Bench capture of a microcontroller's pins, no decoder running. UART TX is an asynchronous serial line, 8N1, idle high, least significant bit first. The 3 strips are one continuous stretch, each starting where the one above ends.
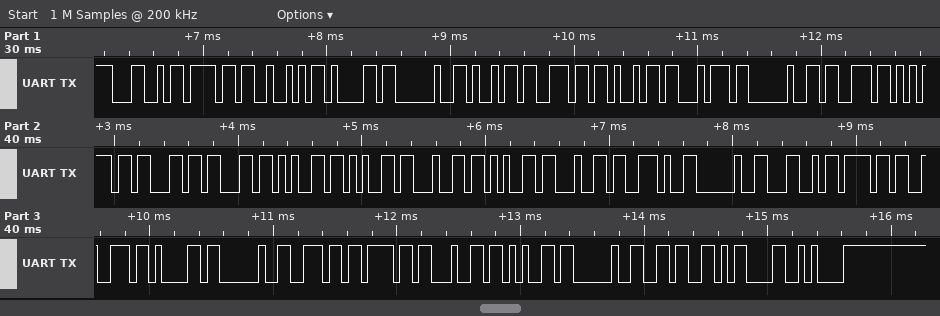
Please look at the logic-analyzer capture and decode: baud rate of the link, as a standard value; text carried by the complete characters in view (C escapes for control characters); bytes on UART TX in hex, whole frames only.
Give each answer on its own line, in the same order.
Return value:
19200 baud
"LoRa init succeeded. Lora node 6\r\n"
4C 6F 52 61 20 69 6E 69 74 20 73 75 63 63 65 65 64 65 64 2E 20 4C 6F 72 61 20 6E 6F 64 65 20 36 0D 0A
